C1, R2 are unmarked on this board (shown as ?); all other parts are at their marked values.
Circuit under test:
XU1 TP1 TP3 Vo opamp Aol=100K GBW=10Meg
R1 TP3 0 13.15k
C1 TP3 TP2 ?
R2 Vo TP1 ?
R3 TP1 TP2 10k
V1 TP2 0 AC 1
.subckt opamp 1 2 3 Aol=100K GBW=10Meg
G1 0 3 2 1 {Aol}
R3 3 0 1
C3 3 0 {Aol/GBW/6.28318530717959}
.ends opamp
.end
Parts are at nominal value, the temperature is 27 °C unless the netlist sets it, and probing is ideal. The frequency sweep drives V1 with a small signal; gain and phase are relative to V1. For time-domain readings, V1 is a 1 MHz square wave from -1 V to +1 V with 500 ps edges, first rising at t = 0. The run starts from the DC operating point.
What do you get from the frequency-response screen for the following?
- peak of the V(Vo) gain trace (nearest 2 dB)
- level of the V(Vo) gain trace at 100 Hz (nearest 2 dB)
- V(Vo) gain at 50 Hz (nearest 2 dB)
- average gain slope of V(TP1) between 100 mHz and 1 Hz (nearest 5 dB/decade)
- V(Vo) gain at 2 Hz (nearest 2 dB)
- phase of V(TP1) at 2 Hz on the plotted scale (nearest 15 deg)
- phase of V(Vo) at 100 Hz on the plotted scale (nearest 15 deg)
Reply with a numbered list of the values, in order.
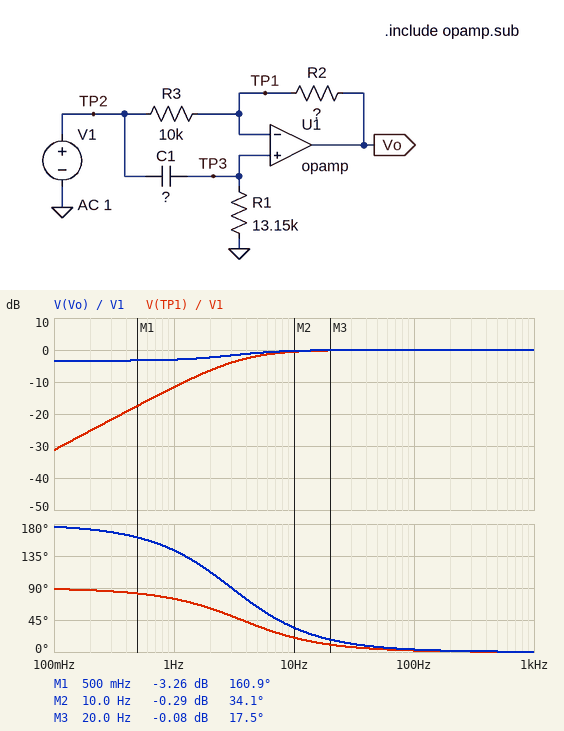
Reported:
1. 0 dB
2. 0 dB
3. 0 dB
4. 20 dB/decade
5. -2 dB
6. 60 deg
7. 0 deg
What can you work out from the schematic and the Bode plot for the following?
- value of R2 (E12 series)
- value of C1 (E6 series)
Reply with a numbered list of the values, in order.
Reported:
1. 6.8 kΩ
2. 3.3 µF
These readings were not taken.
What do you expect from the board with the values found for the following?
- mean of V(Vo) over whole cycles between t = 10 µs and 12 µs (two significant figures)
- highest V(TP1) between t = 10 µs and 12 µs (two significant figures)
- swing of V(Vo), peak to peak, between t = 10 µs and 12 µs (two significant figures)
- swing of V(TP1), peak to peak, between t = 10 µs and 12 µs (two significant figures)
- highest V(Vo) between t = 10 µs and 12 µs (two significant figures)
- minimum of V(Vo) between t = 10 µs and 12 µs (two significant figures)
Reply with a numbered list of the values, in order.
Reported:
1. 1.7 V
2. 2.0 V
3. 2.0 V
4. 2.0 V
5. 2.7 V
6. 680 mV
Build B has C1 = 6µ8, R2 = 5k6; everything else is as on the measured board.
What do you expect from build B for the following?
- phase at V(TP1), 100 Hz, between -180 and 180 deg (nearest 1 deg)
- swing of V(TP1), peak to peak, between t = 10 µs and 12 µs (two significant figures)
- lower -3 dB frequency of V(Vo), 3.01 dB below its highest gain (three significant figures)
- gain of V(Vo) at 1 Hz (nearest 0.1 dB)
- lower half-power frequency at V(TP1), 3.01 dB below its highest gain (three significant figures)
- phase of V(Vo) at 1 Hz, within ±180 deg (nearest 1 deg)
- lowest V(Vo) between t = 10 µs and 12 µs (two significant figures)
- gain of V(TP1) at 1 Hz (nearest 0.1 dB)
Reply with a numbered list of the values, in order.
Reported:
1. 1 deg
2. 2.0 V
3. 1.09 Hz
4. -3.2 dB
5. 1.78 Hz
6. 106 deg
7. 560 mV
8. -6.2 dB
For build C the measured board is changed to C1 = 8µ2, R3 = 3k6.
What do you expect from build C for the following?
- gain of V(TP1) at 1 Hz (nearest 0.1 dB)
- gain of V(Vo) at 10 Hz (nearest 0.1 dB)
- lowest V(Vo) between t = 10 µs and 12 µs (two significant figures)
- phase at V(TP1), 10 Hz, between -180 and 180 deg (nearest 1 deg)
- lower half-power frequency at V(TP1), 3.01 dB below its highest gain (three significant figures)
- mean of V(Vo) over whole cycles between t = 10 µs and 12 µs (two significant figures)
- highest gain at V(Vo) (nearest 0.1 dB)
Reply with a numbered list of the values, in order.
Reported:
1. -5.0 dB
2. 0.2 dB
3. 1.9 V
4. 8 deg
5. 1.48 Hz
6. 2.9 V
7. 5.5 dB
